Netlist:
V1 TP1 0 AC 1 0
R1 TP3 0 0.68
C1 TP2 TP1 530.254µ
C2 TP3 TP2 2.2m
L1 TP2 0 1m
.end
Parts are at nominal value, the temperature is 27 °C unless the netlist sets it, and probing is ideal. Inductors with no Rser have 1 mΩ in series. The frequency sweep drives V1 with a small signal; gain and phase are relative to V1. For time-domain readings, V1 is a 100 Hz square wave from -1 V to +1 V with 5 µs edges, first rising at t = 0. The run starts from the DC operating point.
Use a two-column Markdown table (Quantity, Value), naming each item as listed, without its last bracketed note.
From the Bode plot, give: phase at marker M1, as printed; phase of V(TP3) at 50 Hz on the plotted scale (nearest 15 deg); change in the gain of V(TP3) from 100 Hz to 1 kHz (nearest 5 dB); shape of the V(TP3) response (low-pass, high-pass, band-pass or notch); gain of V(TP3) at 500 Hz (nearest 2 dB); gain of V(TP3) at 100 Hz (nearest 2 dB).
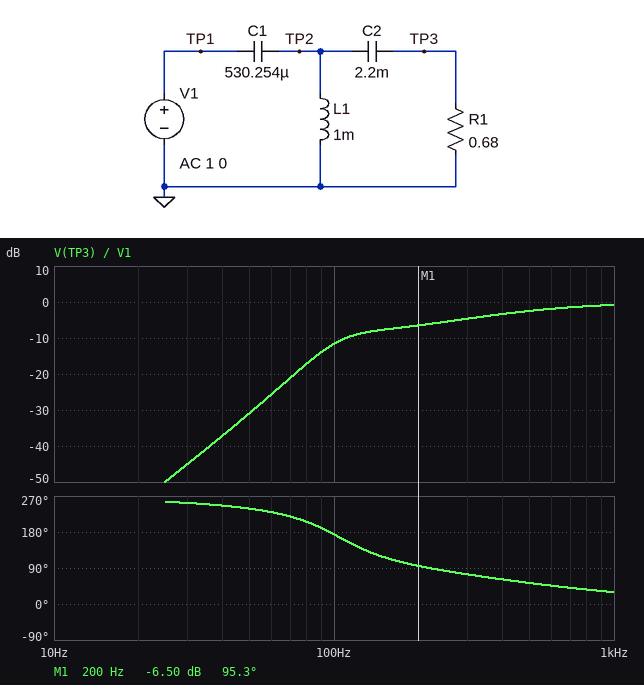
| Quantity | Value |
|---|---|
| phase at marker M1, as printed | 95.3 deg |
| phase of V(TP3) at 50 Hz on the plotted scale | 240 deg |
| change in the gain of V(TP3) from 100 Hz to 1 kHz | 10 dB |
| shape of the V(TP3) response | high-pass |
| gain of V(TP3) at 500 Hz | -2 dB |
| gain of V(TP3) at 100 Hz | -12 dB |
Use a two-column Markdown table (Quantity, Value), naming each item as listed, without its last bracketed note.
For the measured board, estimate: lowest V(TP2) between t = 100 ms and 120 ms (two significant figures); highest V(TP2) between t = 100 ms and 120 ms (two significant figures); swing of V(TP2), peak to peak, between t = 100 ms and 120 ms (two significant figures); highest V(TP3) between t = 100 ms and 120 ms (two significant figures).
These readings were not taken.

| Quantity | Value |
|---|---|
| lowest V(TP2) between t = 100 ms and 120 ms | -2.1 V |
| highest V(TP2) between t = 100 ms and 120 ms | 2.1 V |
| swing of V(TP2), peak to peak, between t = 100 ms and 120 ms | 4.2 V |
| highest V(TP3) between t = 100 ms and 120 ms | 1.9 V |
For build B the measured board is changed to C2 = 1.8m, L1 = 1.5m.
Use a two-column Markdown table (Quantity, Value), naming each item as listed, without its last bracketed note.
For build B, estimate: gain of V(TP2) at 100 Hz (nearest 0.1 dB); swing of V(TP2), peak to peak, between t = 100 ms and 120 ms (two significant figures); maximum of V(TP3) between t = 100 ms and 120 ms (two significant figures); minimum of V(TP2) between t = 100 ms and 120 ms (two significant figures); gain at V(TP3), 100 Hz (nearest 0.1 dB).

| Quantity | Value |
|---|---|
| gain of V(TP2) at 100 Hz | -4.3 dB |
| swing of V(TP2), peak to peak, between t = 100 ms and 120 ms | 4.9 V |
| maximum of V(TP3) between t = 100 ms and 120 ms | 2.1 V |
| minimum of V(TP2) between t = 100 ms and 120 ms | -2.4 V |
| gain at V(TP3), 100 Hz | -8.6 dB |
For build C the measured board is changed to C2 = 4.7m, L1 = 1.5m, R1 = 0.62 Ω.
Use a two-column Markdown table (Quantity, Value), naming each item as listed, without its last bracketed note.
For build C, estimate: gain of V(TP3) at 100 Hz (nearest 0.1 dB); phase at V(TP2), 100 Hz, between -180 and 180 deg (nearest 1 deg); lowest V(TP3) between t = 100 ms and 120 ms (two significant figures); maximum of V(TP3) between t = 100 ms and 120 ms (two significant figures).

| Quantity | Value |
|---|---|
| gain of V(TP3) at 100 Hz | -12.6 dB |
| phase at V(TP2), 100 Hz, between -180 and 180 deg | 92 deg |
| lowest V(TP3) between t = 100 ms and 120 ms | -2.1 V |
| maximum of V(TP3) between t = 100 ms and 120 ms | 2.1 V |
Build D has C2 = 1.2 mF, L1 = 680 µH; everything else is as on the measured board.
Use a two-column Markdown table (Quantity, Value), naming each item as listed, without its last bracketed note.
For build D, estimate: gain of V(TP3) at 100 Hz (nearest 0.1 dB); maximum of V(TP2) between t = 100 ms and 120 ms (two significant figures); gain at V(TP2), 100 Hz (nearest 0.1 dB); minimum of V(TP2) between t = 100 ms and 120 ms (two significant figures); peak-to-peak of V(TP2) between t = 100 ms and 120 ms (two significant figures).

| Quantity | Value |
|---|---|
| gain of V(TP3) at 100 Hz | -19.6 dB |
| maximum of V(TP2) between t = 100 ms and 120 ms | 1.8 V |
| gain at V(TP2), 100 Hz | -12.7 dB |
| minimum of V(TP2) between t = 100 ms and 120 ms | -1.8 V |
| peak-to-peak of V(TP2) between t = 100 ms and 120 ms | 3.6 V |
